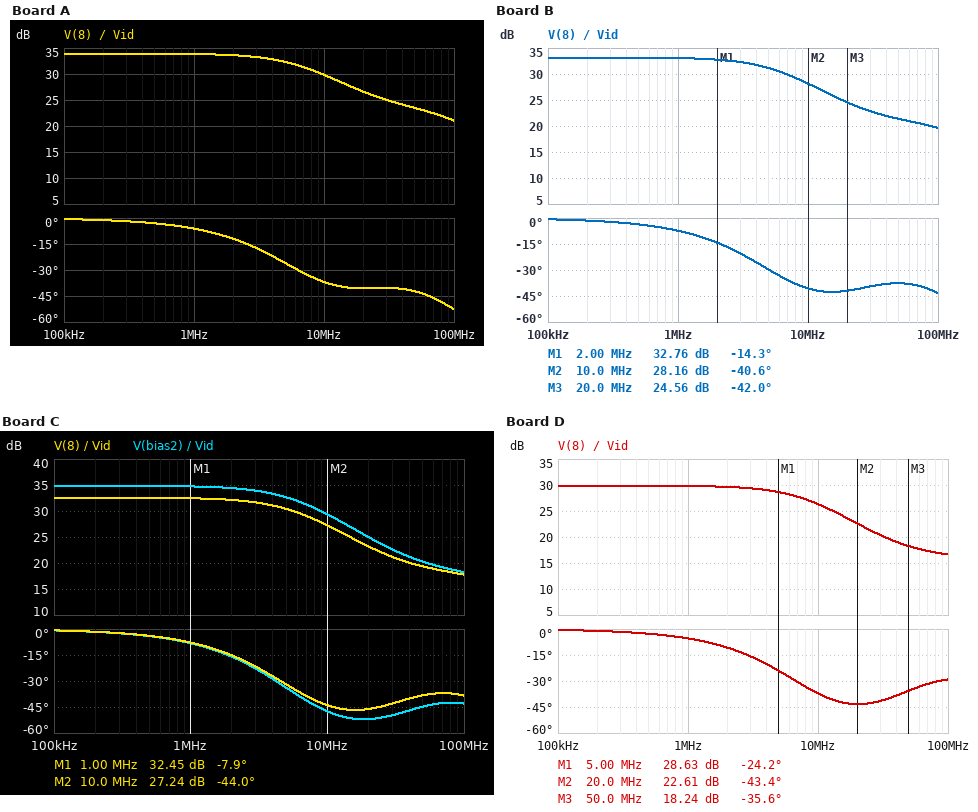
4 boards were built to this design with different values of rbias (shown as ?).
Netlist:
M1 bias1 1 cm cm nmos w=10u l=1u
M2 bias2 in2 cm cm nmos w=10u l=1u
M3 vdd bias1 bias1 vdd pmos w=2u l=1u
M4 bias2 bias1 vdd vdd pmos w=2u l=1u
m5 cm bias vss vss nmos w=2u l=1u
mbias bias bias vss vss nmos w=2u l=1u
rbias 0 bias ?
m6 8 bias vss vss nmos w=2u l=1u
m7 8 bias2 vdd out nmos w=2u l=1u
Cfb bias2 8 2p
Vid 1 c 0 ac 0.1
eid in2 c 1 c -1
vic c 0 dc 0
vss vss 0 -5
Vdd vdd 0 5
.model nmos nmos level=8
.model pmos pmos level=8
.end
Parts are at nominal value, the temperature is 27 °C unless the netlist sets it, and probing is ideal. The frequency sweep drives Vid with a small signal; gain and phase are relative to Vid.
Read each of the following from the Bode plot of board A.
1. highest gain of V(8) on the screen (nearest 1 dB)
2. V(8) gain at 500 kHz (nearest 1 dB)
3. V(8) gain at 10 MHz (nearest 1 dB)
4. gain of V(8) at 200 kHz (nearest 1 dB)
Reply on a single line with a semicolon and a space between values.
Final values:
34 dB; 34 dB; 30 dB; 34 dB
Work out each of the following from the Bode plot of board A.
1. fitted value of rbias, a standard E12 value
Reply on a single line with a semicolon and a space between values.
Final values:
470 kΩ
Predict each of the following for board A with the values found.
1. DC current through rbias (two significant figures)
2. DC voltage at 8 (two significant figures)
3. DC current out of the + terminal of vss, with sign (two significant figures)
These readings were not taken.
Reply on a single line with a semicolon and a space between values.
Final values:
9.9 µA; 3.5 V; -330 µA
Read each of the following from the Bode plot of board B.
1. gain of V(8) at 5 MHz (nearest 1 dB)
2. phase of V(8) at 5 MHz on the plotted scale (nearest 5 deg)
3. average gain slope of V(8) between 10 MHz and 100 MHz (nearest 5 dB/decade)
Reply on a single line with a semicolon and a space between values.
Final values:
31 dB; -30 deg; -10 dB/decade
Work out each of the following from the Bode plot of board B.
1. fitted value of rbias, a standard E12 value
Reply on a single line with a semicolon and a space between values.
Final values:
390 kΩ
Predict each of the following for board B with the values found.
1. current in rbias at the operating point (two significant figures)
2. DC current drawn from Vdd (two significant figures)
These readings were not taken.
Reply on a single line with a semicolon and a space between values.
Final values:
12 µA; 360 µA
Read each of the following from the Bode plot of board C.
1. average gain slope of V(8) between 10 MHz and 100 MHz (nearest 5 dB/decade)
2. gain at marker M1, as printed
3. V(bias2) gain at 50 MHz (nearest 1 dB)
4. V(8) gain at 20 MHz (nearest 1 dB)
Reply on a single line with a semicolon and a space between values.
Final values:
-10 dB/decade; 32.45 dB; 20 dB; 23 dB
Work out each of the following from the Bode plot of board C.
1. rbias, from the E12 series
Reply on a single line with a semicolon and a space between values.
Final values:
330 kΩ
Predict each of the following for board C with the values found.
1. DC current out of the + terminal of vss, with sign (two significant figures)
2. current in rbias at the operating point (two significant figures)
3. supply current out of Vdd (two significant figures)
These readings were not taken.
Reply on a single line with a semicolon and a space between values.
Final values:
-410 µA; 14 µA; 400 µA
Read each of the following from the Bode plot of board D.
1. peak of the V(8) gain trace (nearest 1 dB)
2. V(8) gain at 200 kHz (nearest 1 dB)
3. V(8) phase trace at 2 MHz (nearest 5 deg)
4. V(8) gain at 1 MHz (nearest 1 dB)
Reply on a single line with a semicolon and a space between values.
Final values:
30 dB; 30 dB; -10 deg; 30 dB
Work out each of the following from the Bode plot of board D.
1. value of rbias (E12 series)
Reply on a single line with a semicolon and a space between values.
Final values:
120 kΩ
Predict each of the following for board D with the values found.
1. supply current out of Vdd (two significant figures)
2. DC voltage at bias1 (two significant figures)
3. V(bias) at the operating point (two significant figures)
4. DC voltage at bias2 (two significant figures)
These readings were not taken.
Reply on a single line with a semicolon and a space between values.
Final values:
700 µA; 4.2 V; -4.5 V; 4.2 V
